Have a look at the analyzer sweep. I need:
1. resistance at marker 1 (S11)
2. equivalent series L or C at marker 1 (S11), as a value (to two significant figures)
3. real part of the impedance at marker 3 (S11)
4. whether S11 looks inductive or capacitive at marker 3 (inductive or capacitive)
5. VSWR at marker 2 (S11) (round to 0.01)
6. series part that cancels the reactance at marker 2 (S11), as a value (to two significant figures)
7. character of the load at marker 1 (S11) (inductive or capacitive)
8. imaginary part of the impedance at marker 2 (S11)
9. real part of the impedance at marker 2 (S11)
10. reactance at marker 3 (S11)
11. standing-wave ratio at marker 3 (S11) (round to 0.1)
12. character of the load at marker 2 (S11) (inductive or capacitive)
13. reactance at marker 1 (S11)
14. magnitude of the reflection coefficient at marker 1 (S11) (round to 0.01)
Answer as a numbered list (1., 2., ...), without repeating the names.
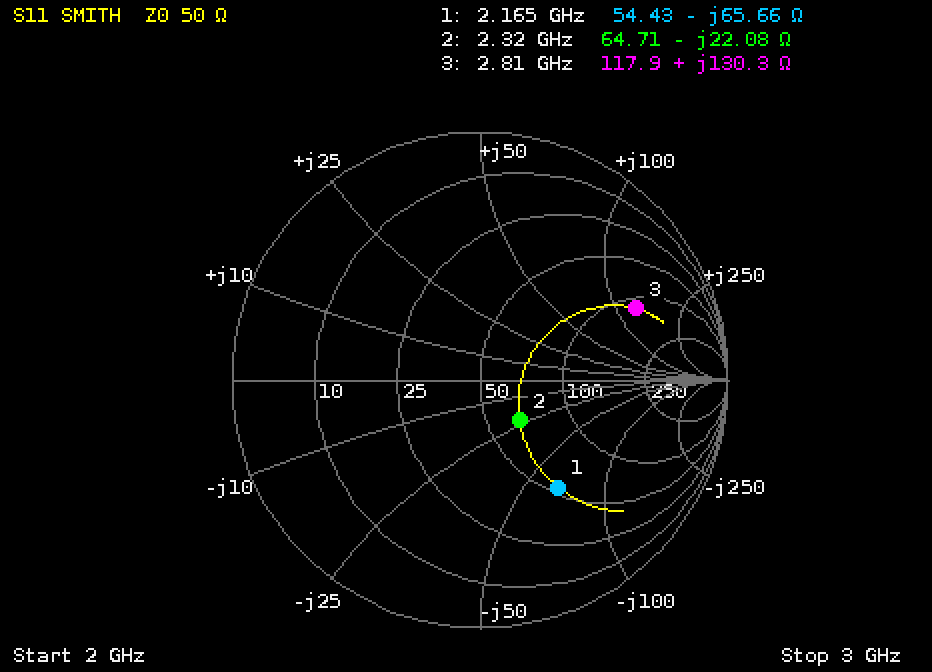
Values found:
1. 54.43 Ω
2. 1.1 pF
3. 117.9 Ω
4. inductive
5. 1.59
6. 1.5 nH
7. capacitive
8. -22.08 Ω
9. 64.71 Ω
10. +130.3 Ω
11. 5.5
12. capacitive
13. -65.66 Ω
14. 0.53
